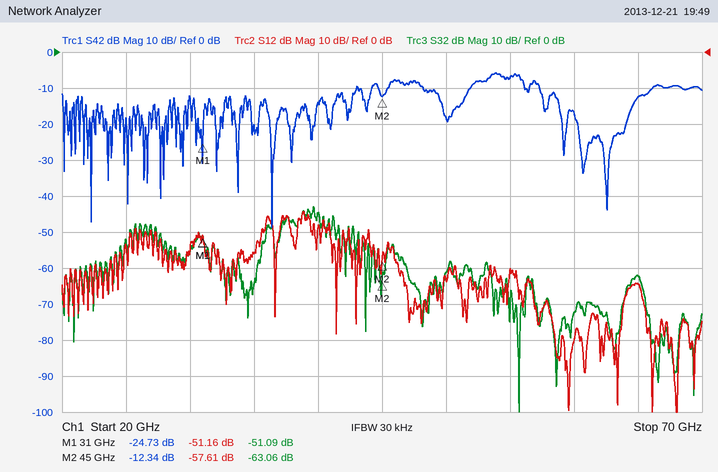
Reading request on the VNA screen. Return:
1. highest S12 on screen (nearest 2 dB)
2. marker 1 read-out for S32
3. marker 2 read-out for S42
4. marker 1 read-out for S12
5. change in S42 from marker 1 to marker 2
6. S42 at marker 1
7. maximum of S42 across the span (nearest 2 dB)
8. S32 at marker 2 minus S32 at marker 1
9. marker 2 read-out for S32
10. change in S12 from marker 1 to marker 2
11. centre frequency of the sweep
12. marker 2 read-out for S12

-44 dB
-51.09 dB
-12.34 dB
-51.16 dB
12.39 dB
-24.73 dB
-6 dB
-11.97 dB
-63.06 dB
-6.45 dB
45 GHz
-57.61 dB
